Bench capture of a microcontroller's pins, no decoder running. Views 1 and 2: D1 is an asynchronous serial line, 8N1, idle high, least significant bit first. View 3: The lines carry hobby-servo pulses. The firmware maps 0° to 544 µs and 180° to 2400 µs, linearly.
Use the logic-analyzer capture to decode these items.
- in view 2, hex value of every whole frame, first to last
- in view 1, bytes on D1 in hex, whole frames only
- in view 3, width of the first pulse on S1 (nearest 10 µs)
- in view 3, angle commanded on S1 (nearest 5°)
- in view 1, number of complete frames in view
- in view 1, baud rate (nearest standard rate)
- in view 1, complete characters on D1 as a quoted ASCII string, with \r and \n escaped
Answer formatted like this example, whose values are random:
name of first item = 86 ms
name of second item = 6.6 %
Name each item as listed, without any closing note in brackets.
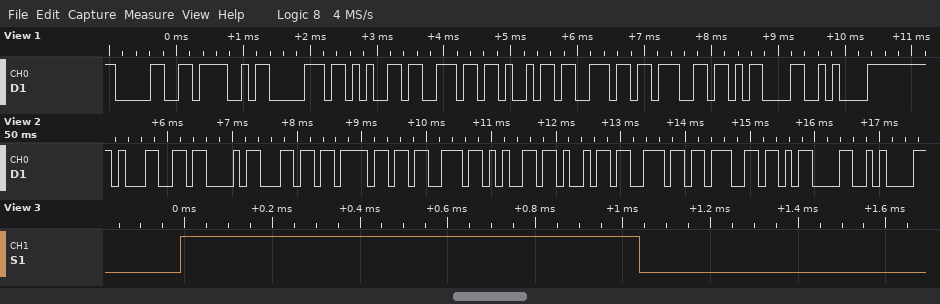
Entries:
in view 2, hex value of every whole frame, first to last = 31 43 6C 6F 73 65 69 6E 67 0D 0A
in view 1, bytes on D1 in hex, whole frames only = 30 4F 70 65 6E 69 6E 67 0D 0A
in view 3, width of the first pulse on S1 = 1050 µs
in view 3, angle commanded on S1 = 50°
in view 1, number of complete frames in view = 10
in view 1, baud rate = 9600 baud
in view 1, complete characters on D1 as a quoted ASCII string, with \r and \n escaped = "0Opening\r\n"
